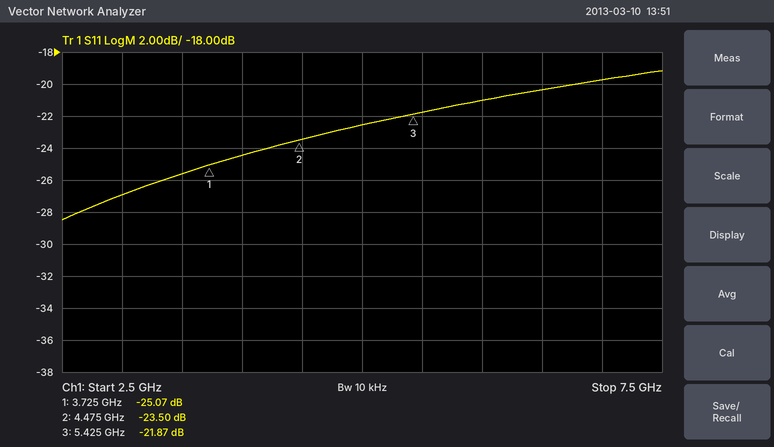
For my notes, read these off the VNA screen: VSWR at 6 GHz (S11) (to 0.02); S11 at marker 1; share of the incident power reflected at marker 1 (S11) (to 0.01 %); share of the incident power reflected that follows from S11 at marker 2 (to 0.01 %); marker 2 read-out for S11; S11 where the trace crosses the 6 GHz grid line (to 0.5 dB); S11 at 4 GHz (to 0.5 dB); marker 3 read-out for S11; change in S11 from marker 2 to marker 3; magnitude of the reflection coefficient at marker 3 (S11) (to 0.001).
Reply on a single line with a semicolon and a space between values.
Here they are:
1.20; -25.07 dB; 0.31 %; 0.45 %; -23.50 dB; -21.0 dB; -24.5 dB; -21.87 dB; 1.63 dB; 0.081
